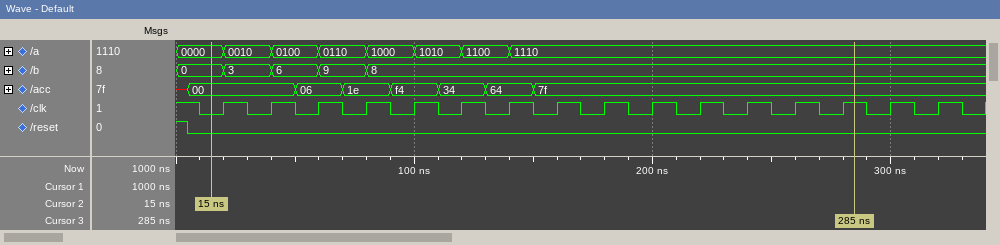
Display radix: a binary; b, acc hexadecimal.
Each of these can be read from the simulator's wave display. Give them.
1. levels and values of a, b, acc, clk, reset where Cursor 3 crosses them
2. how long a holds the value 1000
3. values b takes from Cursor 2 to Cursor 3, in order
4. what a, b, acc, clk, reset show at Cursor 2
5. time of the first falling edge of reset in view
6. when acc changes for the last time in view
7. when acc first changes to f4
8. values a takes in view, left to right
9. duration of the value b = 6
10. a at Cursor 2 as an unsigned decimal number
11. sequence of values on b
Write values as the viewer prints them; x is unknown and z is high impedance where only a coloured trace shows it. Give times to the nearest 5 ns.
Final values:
a=1110, b=8, acc=7f, clk=1, reset=0
20 ns
0, 3, 6, 9, 8
a=0000, b=0, acc=00, clk=0, reset=0
5 ns
150 ns
90 ns
0000, 0010, 0100, 0110, 1000, 1010, 1100, 1110
20 ns
0
0, 3, 6, 9, 8
